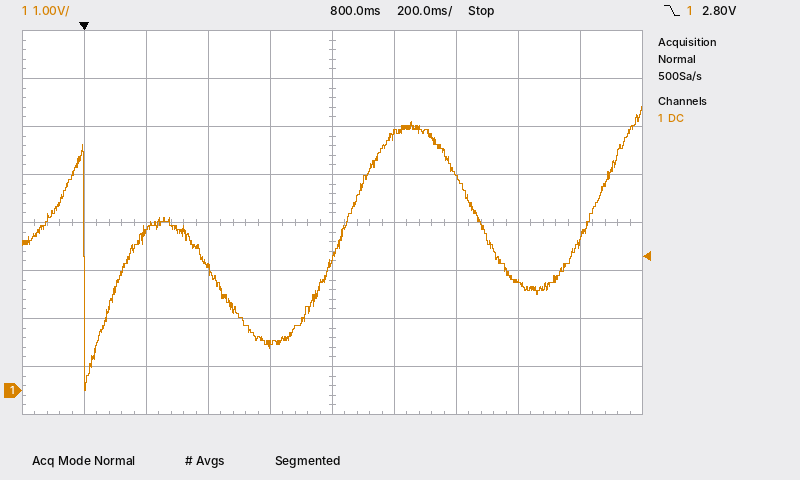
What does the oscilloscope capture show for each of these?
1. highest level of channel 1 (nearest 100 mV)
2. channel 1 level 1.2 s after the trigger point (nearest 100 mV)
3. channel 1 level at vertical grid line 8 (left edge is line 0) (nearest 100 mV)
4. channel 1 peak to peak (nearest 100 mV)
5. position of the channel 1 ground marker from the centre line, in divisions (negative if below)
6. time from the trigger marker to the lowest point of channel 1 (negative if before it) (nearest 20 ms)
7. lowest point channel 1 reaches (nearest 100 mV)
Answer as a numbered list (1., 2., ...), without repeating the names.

1. 5.9 V
2. 4.5 V
3. 2.3 V
4. 5.9 V
5. -3.5 div
6. 0 ms
7. 0.0 V
